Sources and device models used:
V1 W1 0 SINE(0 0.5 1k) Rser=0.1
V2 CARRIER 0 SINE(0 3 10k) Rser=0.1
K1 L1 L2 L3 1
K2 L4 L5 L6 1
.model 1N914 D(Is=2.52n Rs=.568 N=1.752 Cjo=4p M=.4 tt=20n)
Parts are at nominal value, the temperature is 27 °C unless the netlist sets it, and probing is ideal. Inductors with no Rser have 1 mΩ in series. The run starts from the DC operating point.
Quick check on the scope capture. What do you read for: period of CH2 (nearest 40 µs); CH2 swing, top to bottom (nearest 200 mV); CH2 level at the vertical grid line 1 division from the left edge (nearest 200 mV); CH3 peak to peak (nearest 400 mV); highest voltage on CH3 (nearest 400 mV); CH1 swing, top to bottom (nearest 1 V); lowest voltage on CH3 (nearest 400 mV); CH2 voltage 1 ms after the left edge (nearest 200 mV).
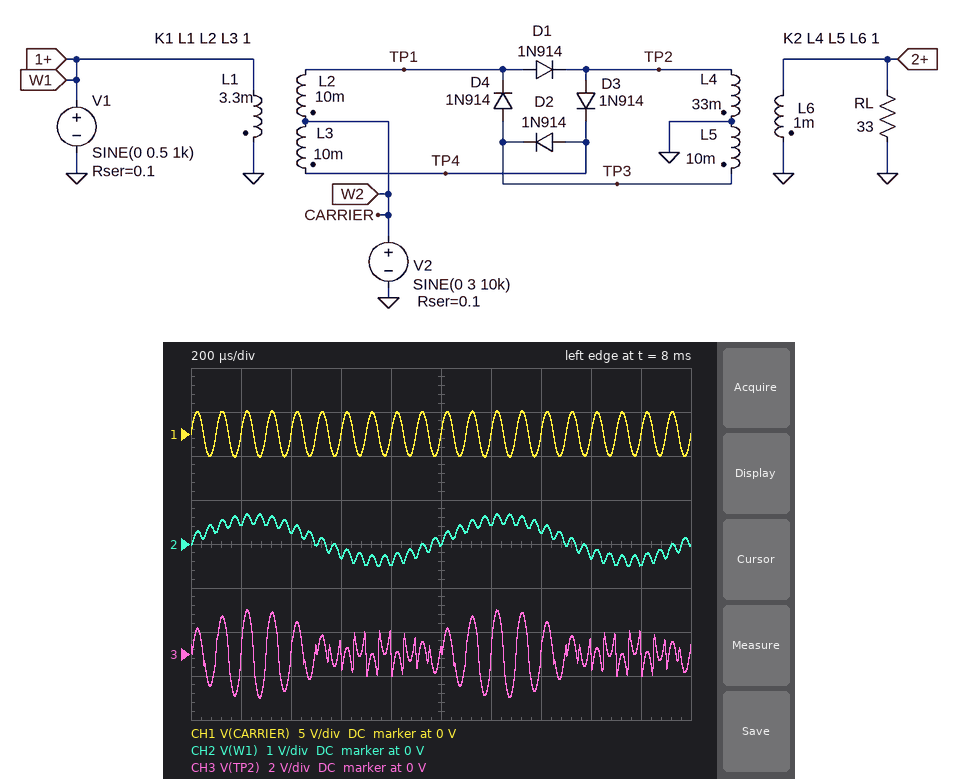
1.00 ms
1.2 V
400 mV
4.0 V
2.0 V
5 V
-2.0 V
0 V
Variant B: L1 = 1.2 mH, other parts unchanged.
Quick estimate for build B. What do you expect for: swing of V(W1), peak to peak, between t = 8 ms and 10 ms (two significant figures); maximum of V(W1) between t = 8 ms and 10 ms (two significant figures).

930 mV
510 mV
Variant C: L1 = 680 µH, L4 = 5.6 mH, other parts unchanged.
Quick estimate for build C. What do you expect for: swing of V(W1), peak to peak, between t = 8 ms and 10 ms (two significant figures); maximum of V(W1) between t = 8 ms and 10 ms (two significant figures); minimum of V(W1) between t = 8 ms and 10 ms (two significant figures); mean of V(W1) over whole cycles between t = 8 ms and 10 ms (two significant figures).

790 mV
370 mV
-420 mV
-45 mV
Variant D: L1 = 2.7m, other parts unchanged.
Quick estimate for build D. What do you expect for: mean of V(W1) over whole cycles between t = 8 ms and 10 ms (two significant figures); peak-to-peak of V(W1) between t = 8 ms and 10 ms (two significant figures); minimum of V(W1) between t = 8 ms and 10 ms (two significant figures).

100 mV
1.2 V
-490 mV
